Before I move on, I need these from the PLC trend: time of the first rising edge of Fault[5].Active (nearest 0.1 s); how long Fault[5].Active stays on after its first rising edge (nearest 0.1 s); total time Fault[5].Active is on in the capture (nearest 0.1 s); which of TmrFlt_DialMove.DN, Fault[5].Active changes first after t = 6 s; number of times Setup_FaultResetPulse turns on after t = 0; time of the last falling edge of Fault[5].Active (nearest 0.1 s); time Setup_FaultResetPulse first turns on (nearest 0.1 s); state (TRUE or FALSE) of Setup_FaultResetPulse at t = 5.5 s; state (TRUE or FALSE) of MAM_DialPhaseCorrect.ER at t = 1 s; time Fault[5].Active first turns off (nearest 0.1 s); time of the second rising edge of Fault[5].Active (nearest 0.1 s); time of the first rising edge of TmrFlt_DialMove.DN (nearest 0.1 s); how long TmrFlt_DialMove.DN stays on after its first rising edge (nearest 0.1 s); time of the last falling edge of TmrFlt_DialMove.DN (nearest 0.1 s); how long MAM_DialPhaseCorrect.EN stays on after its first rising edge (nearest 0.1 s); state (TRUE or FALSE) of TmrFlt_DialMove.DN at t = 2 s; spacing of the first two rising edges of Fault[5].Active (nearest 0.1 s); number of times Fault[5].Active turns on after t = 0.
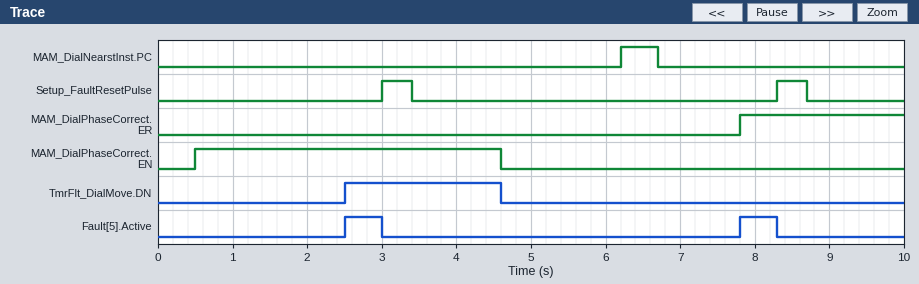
2.5 s
0.5 s
1.0 s
Fault[5].Active
2
8.3 s
3.0 s
FALSE
FALSE
3.0 s
7.8 s
2.5 s
2.1 s
4.6 s
4.1 s
FALSE
5.3 s
2
